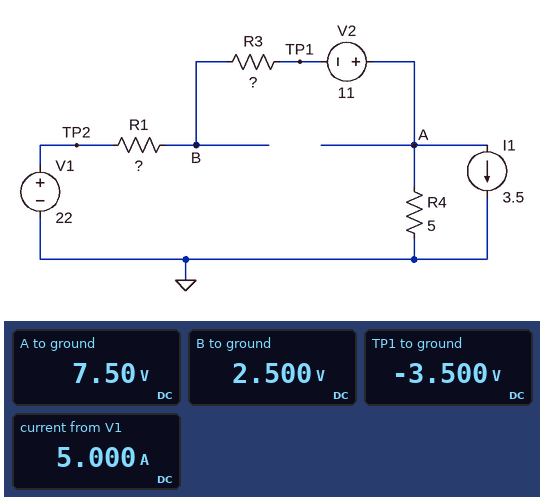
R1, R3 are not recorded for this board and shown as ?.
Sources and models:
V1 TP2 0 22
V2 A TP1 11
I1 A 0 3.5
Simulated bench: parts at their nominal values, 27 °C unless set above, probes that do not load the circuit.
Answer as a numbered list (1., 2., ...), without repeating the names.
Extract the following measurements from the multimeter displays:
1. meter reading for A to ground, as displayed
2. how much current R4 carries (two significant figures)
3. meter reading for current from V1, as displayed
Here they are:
1. 7.50 V
2. 1.5 A
3. 5.000 A
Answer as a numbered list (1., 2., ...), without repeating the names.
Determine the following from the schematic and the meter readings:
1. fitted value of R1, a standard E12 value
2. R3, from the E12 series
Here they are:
1. 3.9 Ω
2. 1.2 Ω
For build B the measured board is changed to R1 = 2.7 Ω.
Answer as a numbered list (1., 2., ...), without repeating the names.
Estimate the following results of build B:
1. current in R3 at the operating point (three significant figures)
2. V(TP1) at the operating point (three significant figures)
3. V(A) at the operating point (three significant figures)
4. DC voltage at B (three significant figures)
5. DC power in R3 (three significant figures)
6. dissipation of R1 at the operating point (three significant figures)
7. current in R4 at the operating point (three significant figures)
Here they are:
1. 5.67 A
2. -129 mV
3. 10.9 V
4. 6.68 V
5. 38.6 W
6. 86.9 W
7. 2.17 A
